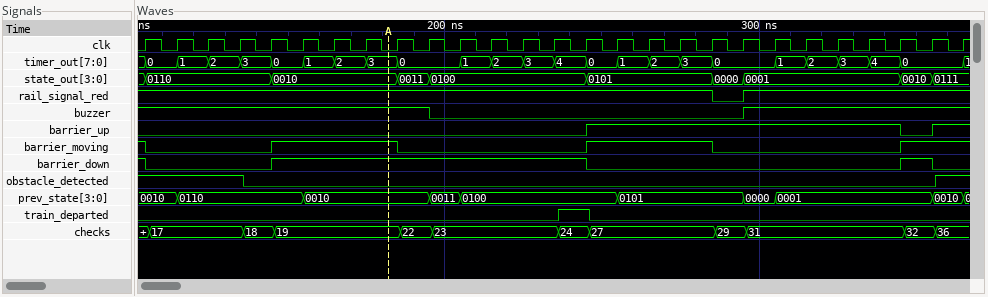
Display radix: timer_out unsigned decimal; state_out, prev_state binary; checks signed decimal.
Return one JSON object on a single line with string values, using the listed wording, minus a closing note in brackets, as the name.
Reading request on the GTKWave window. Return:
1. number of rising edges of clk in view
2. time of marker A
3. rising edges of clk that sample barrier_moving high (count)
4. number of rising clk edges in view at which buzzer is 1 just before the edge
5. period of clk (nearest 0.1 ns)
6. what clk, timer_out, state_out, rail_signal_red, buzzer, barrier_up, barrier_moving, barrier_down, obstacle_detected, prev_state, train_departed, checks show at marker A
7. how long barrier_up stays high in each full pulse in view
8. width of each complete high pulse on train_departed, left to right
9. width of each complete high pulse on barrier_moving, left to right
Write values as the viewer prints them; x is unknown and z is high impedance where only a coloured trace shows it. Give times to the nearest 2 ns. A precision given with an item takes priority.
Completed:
{"number of rising edges of clk in view": "27", "time of marker A": "182 ns", "rising edges of clk that sample barrier_moving high": "11", "number of rising clk edges in view at which buzzer is 1 just before the edge": "17", "period of clk": "10 ns", "what clk, timer_out, state_out, rail_signal_red, buzzer, barrier_up, barrier_moving, barrier_down, obstacle_detected, prev_state, train_departed, checks show at marker A": "clk=0, timer_out=3, state_out=0010, rail_signal_red=1, buzzer=1, barrier_up=0, barrier_moving=1, barrier_down=1, obstacle_detected=0, prev_state=0010, train_departed=0, checks=19", "how long barrier_up stays high in each full pulse in view": "100 ns", "width of each complete high pulse on train_departed, left to right": "10 ns", "width of each complete high pulse on barrier_moving, left to right": "40 ns, 40 ns"}
